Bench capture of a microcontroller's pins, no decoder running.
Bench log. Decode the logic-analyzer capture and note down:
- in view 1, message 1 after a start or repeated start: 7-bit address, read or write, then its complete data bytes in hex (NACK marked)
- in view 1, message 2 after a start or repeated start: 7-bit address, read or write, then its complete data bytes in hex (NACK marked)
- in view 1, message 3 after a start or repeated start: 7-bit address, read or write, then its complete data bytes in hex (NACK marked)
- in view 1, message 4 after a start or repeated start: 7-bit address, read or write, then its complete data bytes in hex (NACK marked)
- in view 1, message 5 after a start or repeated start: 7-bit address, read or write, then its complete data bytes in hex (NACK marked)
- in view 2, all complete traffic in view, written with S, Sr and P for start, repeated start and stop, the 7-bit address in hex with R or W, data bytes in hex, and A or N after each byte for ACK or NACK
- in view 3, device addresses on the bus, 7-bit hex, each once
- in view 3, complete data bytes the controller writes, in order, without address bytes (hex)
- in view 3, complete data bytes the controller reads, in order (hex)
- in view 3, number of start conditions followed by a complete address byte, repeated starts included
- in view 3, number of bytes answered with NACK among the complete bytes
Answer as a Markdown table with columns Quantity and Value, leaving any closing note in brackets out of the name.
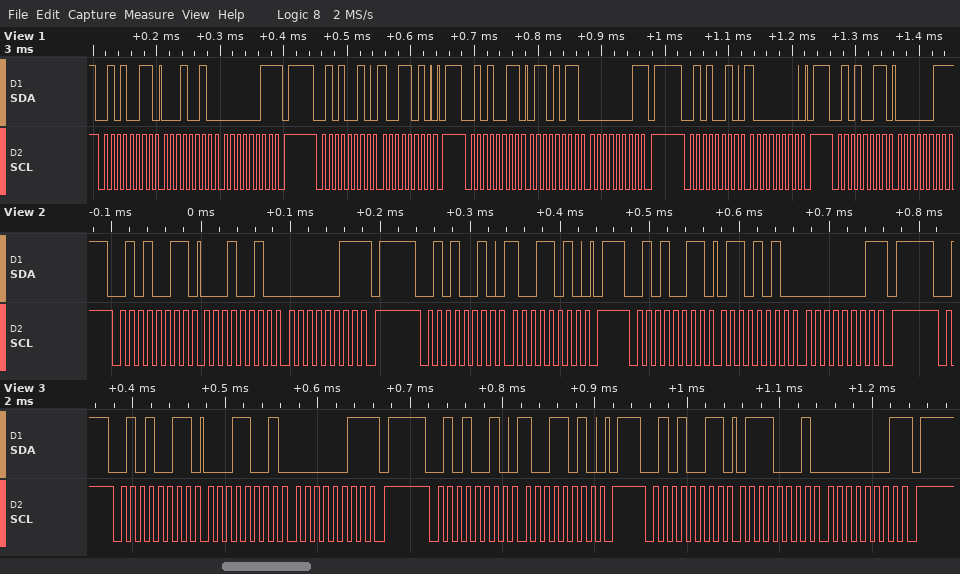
| Quantity | Value |
|---|---|
| in view 1, message 1 after a start or repeated start: 7-bit address, read or write, then its complete data bytes in hex | 0x29 read: 12 03 NACK |
| in view 1, message 2 after a start or repeated start: 7-bit address, read or write, then its complete data bytes in hex | 0x29 write: 9A |
| in view 1, message 3 after a start or repeated start: 7-bit address, read or write, then its complete data bytes in hex | 0x29 read: 6B 01 NACK |
| in view 1, message 4 after a start or repeated start: 7-bit address, read or write, then its complete data bytes in hex | 0x29 write: 80 |
| in view 1, message 5 after a start or repeated start: 7-bit address, read or write, then its complete data bytes in hex | 0x29 read: 03 NACK |
| in view 2, all complete traffic in view, written with S, Sr and P for start, repeated start and stop, the 7-bit address in hex with R or W, data bytes in hex, and A or N after each byte for ACK or NACK | S 29R A 12 A 03 N P S 29W A 9A A P S 29R A 6A A 01 N P |
| in view 3, device addresses on the bus, 7-bit hex, each once | 0x29 |
| in view 3, complete data bytes the controller writes, in order, without address bytes | 9A |
| in view 3, complete data bytes the controller reads, in order | 19 03 71 01 |
| in view 3, number of start conditions followed by a complete address byte, repeated starts included | 3 |
| in view 3, number of bytes answered with NACK among the complete bytes | 2 |
